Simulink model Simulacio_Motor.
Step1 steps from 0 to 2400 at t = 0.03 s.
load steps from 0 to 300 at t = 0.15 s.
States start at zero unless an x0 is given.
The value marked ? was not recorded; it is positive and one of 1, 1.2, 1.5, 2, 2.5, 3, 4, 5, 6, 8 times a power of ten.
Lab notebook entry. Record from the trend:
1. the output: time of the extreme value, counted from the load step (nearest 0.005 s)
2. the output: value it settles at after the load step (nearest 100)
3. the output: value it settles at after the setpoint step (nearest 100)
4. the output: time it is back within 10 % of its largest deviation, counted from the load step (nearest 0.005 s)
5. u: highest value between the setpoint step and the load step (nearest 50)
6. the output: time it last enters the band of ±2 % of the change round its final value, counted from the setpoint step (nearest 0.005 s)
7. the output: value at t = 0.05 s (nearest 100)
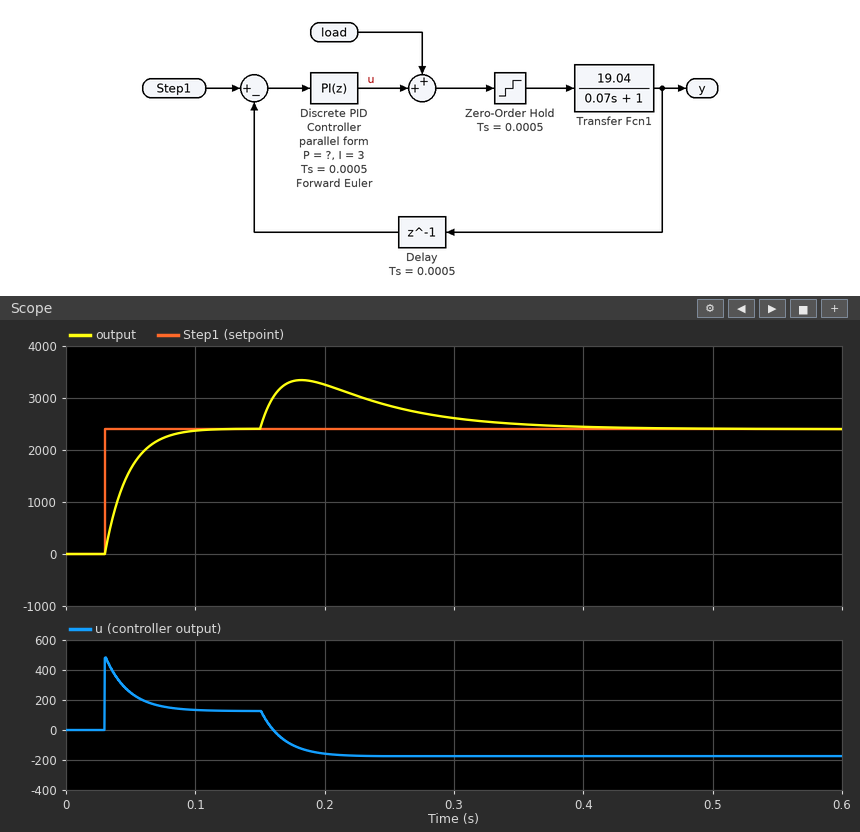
0.030 s
2400
2400
0.205 s
500
0.065 s
1600
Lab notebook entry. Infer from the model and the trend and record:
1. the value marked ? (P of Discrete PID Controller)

0.2
